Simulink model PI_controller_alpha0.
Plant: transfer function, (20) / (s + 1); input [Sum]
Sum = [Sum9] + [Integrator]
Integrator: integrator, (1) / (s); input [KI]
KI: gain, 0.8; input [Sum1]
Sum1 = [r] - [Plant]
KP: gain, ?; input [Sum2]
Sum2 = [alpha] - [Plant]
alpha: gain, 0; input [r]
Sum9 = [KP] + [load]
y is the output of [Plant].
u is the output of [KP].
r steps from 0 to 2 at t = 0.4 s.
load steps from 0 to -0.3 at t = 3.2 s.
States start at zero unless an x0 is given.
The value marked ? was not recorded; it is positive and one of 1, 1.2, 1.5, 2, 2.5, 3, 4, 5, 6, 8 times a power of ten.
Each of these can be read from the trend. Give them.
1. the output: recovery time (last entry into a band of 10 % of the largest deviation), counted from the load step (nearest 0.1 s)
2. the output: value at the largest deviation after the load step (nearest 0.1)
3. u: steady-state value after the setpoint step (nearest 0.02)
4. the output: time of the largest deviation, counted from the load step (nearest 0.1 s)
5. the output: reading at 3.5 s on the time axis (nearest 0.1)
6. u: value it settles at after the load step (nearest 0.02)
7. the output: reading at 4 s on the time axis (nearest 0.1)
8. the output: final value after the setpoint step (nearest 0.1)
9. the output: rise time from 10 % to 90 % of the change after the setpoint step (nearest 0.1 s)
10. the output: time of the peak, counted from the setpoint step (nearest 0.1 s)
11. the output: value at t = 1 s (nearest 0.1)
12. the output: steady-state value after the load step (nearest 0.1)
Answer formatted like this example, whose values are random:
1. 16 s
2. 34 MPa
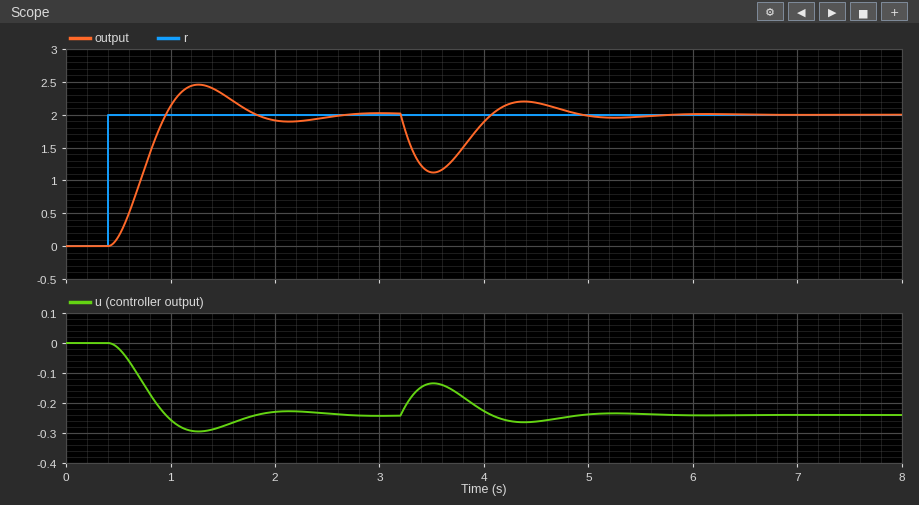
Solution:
1. 1.5 s
2. 1.1
3. -0.24
4. 0.3 s
5. 1.1
6. -0.24
7. 1.9
8. 2.0
9. 0.4 s
10. 0.9 s
11. 2.1
12. 2.0
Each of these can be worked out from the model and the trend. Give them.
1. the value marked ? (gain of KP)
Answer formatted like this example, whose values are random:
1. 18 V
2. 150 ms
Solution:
1. 0.12
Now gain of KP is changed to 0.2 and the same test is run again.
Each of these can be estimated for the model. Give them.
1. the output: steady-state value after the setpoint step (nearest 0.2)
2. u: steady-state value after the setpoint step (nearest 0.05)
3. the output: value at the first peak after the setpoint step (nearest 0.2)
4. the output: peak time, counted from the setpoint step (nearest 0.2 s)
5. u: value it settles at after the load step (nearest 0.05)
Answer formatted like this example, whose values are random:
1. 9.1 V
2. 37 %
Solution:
1. 2.0
2. -0.40
3. 2.2
4. 1.0 s
5. -0.40
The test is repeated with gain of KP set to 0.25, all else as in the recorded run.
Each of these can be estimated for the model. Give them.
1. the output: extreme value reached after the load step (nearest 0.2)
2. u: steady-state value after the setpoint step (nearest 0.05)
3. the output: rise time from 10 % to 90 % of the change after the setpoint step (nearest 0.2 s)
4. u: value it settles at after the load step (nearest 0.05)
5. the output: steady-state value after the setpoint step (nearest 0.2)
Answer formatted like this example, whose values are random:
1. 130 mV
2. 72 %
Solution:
1. 1.4
2. -0.50
3. 0.6 s
4. -0.50
5. 2.0
